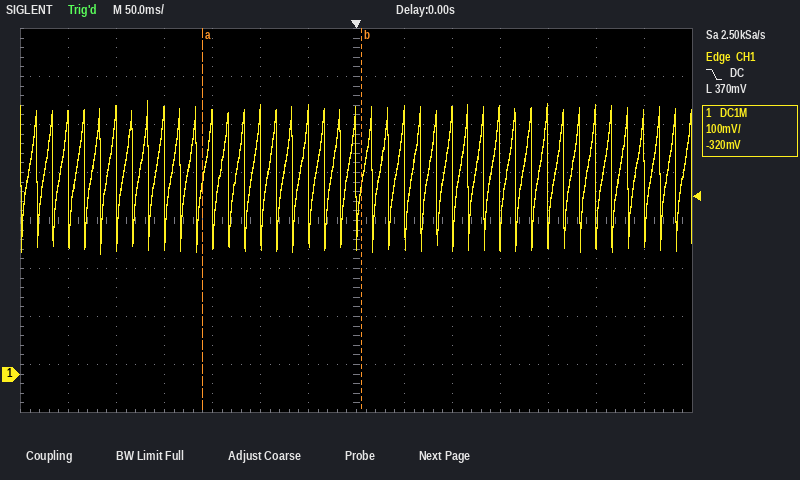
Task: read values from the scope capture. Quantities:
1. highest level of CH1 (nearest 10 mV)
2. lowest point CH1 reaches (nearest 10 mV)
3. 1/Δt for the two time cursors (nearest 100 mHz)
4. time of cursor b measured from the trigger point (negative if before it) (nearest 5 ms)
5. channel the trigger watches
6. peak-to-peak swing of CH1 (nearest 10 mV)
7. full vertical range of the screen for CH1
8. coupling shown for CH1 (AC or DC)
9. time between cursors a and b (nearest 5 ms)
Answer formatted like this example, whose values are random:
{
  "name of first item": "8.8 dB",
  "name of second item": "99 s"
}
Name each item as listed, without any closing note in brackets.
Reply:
{
  "highest level of CH1": "570 mV",
  "lowest point CH1 reaches": "250 mV",
  "1/Δt for the two time cursors": "6.1 Hz",
  "time of cursor b measured from the trigger point (negative if before it)": "+5 ms",
  "channel the trigger watches": "CH1",
  "peak-to-peak swing of CH1": "320 mV",
  "full vertical range of the screen for CH1": "800 mV",
  "coupling shown for CH1": "DC",
  "time between cursors a and b": "165 ms"
}
